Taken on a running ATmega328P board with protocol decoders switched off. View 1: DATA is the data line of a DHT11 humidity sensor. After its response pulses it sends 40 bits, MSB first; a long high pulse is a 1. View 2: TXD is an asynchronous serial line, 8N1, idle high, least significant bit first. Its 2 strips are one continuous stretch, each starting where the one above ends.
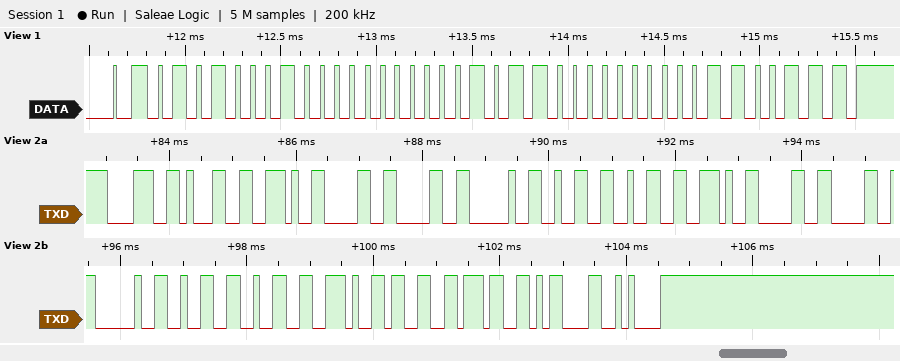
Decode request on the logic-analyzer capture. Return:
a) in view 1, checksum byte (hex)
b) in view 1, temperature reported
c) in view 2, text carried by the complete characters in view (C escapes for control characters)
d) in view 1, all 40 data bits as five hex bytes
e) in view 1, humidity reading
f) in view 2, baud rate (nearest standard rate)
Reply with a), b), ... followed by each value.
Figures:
a) 0x67
b) 22.0 °C
c) "81.00 22.00 22.37\r\n"
d) 51 00 16 00 67
e) 81 %
f) 9600 baud
